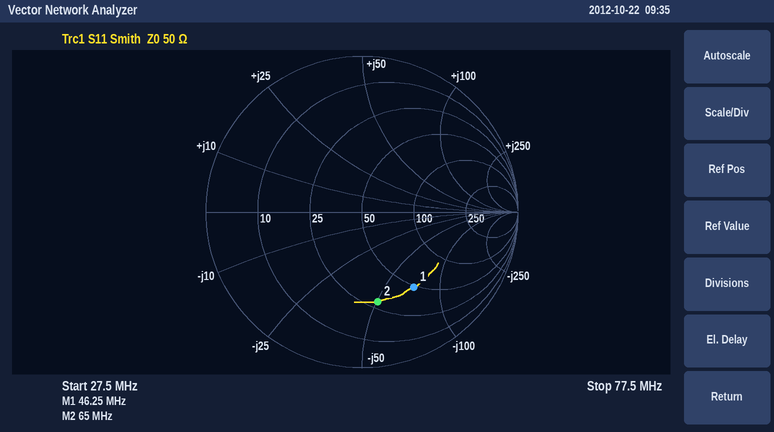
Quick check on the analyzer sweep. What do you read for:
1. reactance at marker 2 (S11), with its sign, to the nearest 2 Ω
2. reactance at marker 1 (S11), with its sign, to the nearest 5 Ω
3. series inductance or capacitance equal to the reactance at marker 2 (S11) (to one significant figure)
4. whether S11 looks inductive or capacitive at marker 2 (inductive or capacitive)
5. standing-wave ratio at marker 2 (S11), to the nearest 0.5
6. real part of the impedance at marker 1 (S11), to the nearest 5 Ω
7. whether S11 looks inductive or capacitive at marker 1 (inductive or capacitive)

-50 Ω
-70 Ω
50 pF
capacitive
4.0
50 Ω
capacitive
